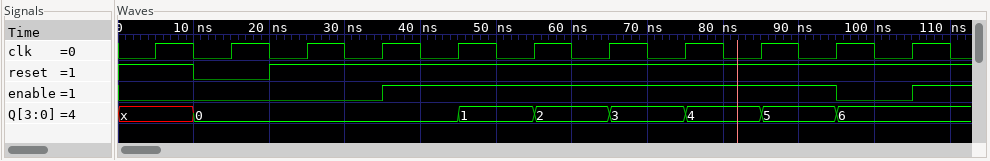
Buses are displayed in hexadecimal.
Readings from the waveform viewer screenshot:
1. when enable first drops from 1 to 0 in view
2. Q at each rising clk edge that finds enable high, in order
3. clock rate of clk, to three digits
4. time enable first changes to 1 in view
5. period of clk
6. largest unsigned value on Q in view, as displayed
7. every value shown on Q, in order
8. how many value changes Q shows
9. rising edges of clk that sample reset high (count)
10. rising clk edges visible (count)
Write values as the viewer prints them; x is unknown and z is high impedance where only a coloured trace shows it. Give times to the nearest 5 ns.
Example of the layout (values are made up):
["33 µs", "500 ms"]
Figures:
["95 ns", "0, 1, 2, 3, 4, 5", "100 MHz", "35 ns", "10 ns", "6", "x, 0, 1, 2, 3, 4, 5, 6", "7", "10", "11"]
